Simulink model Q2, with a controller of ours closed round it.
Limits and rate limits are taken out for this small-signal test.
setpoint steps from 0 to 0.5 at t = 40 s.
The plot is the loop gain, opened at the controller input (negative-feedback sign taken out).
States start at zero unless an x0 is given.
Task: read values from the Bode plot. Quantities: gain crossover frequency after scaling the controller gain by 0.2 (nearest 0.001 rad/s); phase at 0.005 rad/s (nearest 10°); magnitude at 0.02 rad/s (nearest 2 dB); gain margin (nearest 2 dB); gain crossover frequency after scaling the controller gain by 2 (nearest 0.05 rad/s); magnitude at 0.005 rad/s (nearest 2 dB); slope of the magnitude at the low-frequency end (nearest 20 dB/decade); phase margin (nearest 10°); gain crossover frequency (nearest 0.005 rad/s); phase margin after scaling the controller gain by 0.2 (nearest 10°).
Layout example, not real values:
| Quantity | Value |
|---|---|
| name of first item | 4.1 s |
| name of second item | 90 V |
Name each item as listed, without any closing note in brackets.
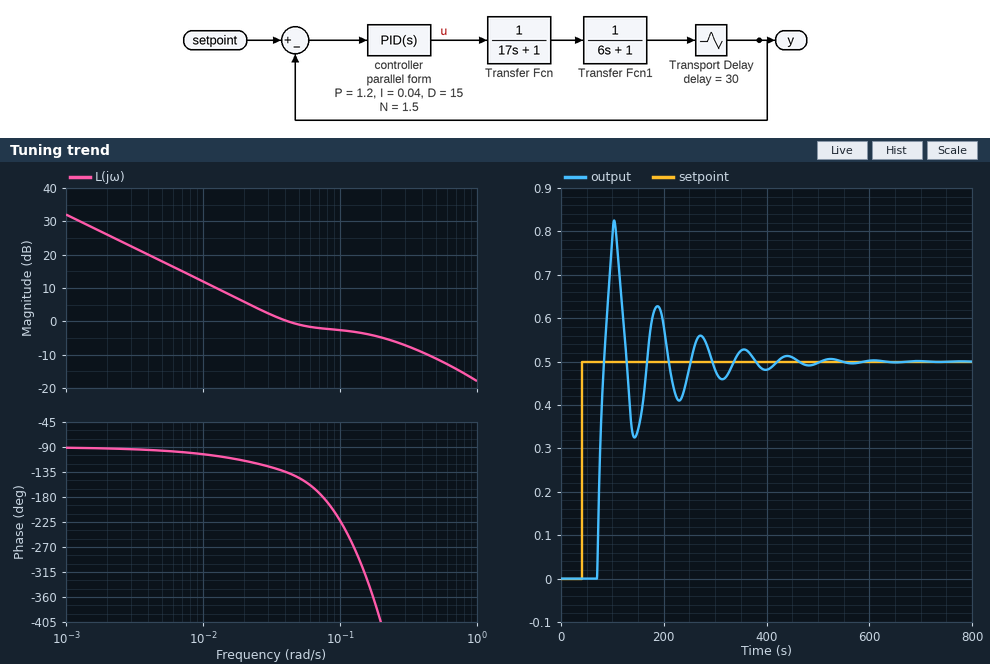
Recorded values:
| Quantity | Value |
|---|---|
| gain crossover frequency after scaling the controller gain by 0.2 | 0.008 rad/s |
| phase at 0.005 rad/s | -100° |
| magnitude at 0.02 rad/s | 6 dB |
| gain margin | 2 dB |
| gain crossover frequency after scaling the controller gain by 2 | 0.25 rad/s |
| magnitude at 0.005 rad/s | 18 dB |
| slope of the magnitude at the low-frequency end | -20 dB/decade |
| phase margin | 40° |
| gain crossover frequency | 0.040 rad/s |
| phase margin after scaling the controller gain by 0.2 | 80° |
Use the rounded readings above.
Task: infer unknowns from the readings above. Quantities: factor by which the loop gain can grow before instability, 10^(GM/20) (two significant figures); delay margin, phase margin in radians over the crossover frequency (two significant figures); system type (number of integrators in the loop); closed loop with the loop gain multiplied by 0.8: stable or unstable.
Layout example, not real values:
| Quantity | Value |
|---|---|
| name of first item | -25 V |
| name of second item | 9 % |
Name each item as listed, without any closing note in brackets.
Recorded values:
| Quantity | Value |
|---|---|
| factor by which the loop gain can grow before instability, 10^(GM/20) | 1.3 |
| delay margin, phase margin in radians over the crossover frequency | 17 s |
| system type | 1 |
| closed loop with the loop gain multiplied by 0.8: stable or unstable | stable |
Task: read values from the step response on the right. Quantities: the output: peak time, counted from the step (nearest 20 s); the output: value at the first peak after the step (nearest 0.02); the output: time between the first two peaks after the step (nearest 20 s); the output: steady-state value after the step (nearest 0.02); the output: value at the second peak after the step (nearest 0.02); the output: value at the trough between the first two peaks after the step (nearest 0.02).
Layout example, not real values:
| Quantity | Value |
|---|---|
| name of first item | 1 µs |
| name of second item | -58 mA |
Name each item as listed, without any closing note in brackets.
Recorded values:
| Quantity | Value |
|---|---|
| the output: peak time, counted from the step | 60 s |
| the output: value at the first peak after the step | 0.82 |
| the output: time between the first two peaks after the step | 80 s |
| the output: steady-state value after the step | 0.50 |
| the output: value at the second peak after the step | 0.62 |
| the output: value at the trough between the first two peaks after the step | 0.32 |
